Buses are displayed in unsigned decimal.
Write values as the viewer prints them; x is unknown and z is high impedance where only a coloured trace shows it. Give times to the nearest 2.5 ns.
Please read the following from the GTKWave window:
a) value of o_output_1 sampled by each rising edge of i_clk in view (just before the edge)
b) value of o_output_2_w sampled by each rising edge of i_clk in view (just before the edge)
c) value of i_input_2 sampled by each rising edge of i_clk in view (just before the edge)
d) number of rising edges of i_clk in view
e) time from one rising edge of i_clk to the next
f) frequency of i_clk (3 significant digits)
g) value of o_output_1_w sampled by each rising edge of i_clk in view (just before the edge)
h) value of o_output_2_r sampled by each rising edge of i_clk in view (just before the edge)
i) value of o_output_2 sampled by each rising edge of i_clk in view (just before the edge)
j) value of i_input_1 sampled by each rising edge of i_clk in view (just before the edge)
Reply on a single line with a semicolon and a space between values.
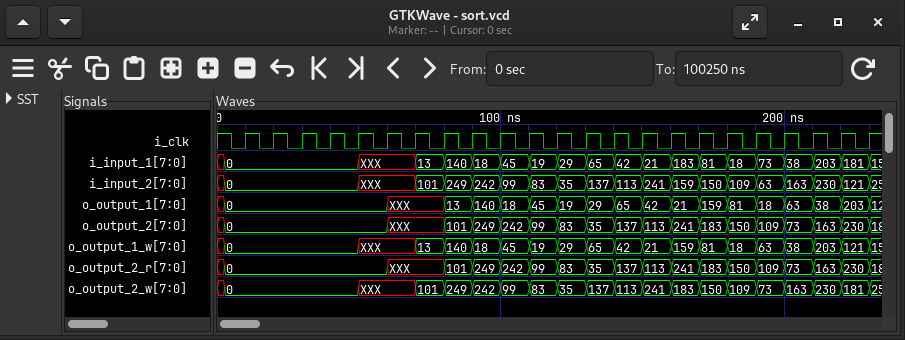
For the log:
0, 0, 0, 0, 0, 0, XXX, XXX, 13, 140, 18, 45, 19, 29, 65, 42, 21, 159, 81, 18, 63, 38, 203; 0, 0, 0, 0, 0, XXX, XXX, 101, 249, 242, 99, 83, 35, 137, 113, 241, 183, 150, 109, 73, 163, 230, 181; 0, 0, 0, 0, 0, XXX, XXX, 101, 249, 242, 99, 83, 35, 137, 113, 241, 159, 150, 109, 63, 163, 230, 121; 23; 10 ns; 100 MHz; 0, 0, 0, 0, 0, XXX, XXX, 13, 140, 18, 45, 19, 29, 65, 42, 21, 159, 81, 18, 63, 38, 203, 121; 0, 0, 0, 0, 0, 0, XXX, XXX, 101, 249, 242, 99, 83, 35, 137, 113, 241, 183, 150, 109, 73, 163, 230; 0, 0, 0, 0, 0, 0, XXX, XXX, 101, 249, 242, 99, 83, 35, 137, 113, 241, 183, 150, 109, 73, 163, 230; 0, 0, 0, 0, 0, XXX, XXX, 13, 140, 18, 45, 19, 29, 65, 42, 21, 183, 81, 18, 73, 38, 203, 181
